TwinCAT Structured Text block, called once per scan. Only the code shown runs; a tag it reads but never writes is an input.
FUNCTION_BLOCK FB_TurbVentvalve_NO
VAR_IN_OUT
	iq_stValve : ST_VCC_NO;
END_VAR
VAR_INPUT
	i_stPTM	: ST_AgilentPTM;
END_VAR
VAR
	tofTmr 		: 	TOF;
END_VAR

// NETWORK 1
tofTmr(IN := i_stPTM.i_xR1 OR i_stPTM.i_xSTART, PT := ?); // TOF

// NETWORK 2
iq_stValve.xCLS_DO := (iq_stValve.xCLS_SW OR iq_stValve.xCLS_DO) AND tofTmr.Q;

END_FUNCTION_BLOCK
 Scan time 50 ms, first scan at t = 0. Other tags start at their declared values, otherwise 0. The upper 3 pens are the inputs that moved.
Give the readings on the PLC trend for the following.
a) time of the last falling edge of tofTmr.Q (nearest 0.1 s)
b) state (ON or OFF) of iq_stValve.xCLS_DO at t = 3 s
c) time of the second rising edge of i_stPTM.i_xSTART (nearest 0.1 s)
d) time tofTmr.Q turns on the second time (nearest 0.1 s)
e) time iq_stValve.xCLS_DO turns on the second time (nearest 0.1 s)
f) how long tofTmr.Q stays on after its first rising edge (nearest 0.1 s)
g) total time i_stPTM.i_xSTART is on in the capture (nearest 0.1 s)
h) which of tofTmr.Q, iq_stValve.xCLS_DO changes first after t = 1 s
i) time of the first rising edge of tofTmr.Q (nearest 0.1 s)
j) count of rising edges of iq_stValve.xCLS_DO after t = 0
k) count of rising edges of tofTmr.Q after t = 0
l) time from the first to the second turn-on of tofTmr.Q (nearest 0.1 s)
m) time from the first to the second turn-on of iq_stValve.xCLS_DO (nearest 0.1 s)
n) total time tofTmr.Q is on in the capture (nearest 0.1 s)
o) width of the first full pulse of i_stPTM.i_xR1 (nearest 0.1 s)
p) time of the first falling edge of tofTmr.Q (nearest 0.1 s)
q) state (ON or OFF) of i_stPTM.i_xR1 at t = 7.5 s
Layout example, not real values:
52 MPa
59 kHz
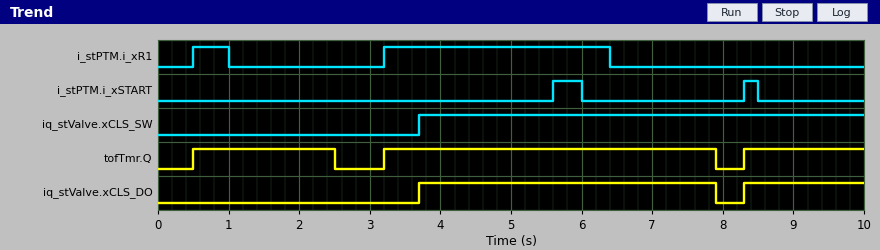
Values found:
7.9 s
OFF
8.3 s
3.2 s
8.3 s
2.0 s
0.6 s
tofTmr.Q
0.5 s
2
3
2.7 s
4.6 s
8.4 s
0.5 s
2.5 s
OFF
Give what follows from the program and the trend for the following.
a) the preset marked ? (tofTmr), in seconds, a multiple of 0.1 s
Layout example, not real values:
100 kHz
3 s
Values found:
1.5 s
